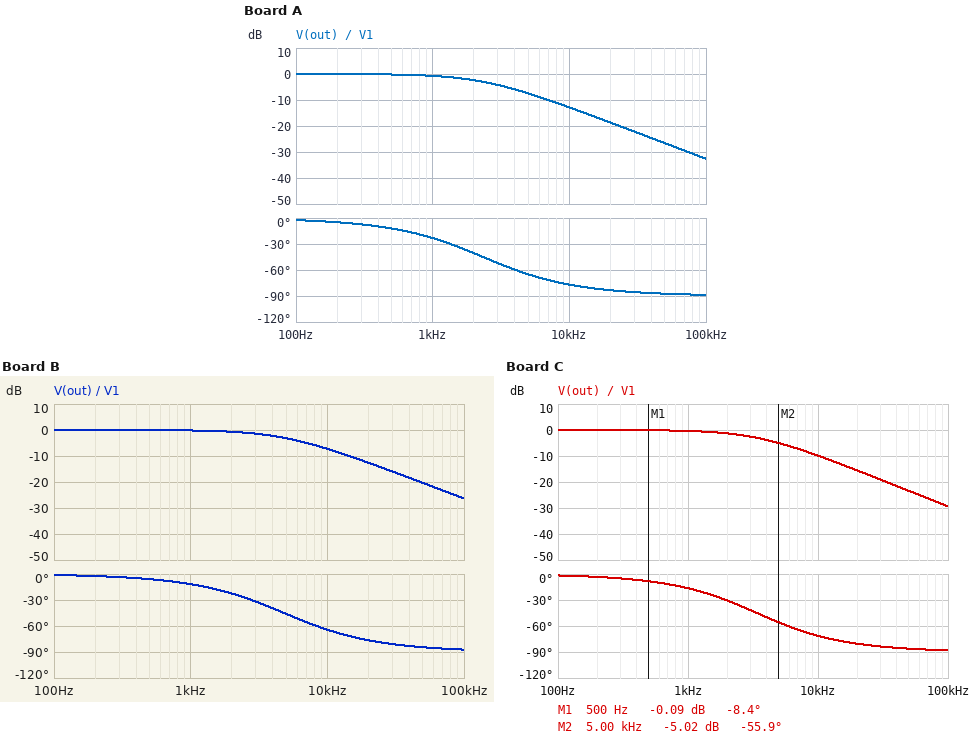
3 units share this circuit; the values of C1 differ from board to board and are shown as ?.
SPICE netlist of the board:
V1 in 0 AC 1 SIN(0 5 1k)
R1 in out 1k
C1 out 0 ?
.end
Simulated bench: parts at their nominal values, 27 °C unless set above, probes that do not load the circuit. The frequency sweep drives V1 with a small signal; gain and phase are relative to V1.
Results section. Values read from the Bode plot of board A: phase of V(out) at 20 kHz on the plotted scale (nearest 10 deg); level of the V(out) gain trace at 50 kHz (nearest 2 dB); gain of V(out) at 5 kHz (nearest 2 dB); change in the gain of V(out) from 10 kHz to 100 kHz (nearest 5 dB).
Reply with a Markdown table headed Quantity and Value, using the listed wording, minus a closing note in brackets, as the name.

| Quantity | Value |
|---|---|
| phase of V(out) at 20 kHz on the plotted scale | -80 deg |
| level of the V(out) gain trace at 50 kHz | -26 dB |
| gain of V(out) at 5 kHz | -8 dB |
| change in the gain of V(out) from 10 kHz to 100 kHz | -20 dB |
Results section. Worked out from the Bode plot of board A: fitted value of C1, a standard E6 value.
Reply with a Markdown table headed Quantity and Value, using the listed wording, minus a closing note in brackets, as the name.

| Quantity | Value |
|---|---|
| fitted value of C1, a standard E6 value | 68 nF |
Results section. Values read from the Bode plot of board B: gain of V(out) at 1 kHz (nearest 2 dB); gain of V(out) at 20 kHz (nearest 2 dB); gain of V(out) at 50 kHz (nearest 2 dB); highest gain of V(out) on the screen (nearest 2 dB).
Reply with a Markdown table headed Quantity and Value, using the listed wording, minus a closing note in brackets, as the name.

| Quantity | Value |
|---|---|
| gain of V(out) at 1 kHz | 0 dB |
| gain of V(out) at 20 kHz | -12 dB |
| gain of V(out) at 50 kHz | -20 dB |
| highest gain of V(out) on the screen | 0 dB |
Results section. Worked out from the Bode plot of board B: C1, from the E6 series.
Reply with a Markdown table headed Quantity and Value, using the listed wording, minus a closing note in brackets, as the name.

| Quantity | Value |
|---|---|
| C1, from the E6 series | 33 nF |
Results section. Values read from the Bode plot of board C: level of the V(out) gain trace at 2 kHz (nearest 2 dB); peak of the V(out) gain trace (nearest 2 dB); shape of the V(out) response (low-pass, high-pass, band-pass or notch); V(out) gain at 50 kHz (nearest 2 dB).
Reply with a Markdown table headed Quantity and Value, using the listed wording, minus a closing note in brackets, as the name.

| Quantity | Value |
|---|---|
| level of the V(out) gain trace at 2 kHz | -2 dB |
| peak of the V(out) gain trace | 0 dB |
| shape of the V(out) response | low-pass |
| V(out) gain at 50 kHz | -24 dB |
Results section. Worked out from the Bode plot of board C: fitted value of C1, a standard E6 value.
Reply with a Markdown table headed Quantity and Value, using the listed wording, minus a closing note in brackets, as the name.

| Quantity | Value |
|---|---|
| fitted value of C1, a standard E6 value | 47 nF |
